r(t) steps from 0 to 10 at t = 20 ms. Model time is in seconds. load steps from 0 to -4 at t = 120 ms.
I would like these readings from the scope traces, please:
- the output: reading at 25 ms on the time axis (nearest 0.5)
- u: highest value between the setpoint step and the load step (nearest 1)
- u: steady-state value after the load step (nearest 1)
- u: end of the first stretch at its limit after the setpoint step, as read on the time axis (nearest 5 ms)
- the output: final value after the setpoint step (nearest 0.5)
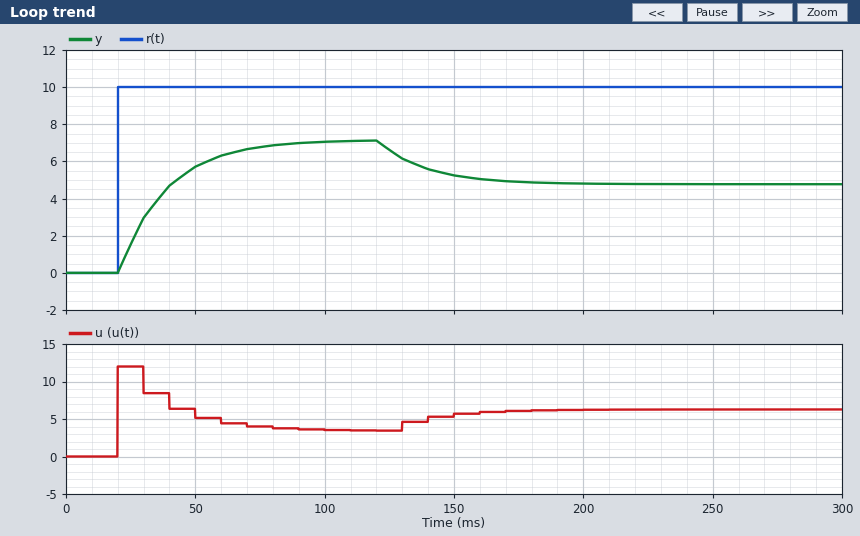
1.5
12
6
30 ms
7.0
